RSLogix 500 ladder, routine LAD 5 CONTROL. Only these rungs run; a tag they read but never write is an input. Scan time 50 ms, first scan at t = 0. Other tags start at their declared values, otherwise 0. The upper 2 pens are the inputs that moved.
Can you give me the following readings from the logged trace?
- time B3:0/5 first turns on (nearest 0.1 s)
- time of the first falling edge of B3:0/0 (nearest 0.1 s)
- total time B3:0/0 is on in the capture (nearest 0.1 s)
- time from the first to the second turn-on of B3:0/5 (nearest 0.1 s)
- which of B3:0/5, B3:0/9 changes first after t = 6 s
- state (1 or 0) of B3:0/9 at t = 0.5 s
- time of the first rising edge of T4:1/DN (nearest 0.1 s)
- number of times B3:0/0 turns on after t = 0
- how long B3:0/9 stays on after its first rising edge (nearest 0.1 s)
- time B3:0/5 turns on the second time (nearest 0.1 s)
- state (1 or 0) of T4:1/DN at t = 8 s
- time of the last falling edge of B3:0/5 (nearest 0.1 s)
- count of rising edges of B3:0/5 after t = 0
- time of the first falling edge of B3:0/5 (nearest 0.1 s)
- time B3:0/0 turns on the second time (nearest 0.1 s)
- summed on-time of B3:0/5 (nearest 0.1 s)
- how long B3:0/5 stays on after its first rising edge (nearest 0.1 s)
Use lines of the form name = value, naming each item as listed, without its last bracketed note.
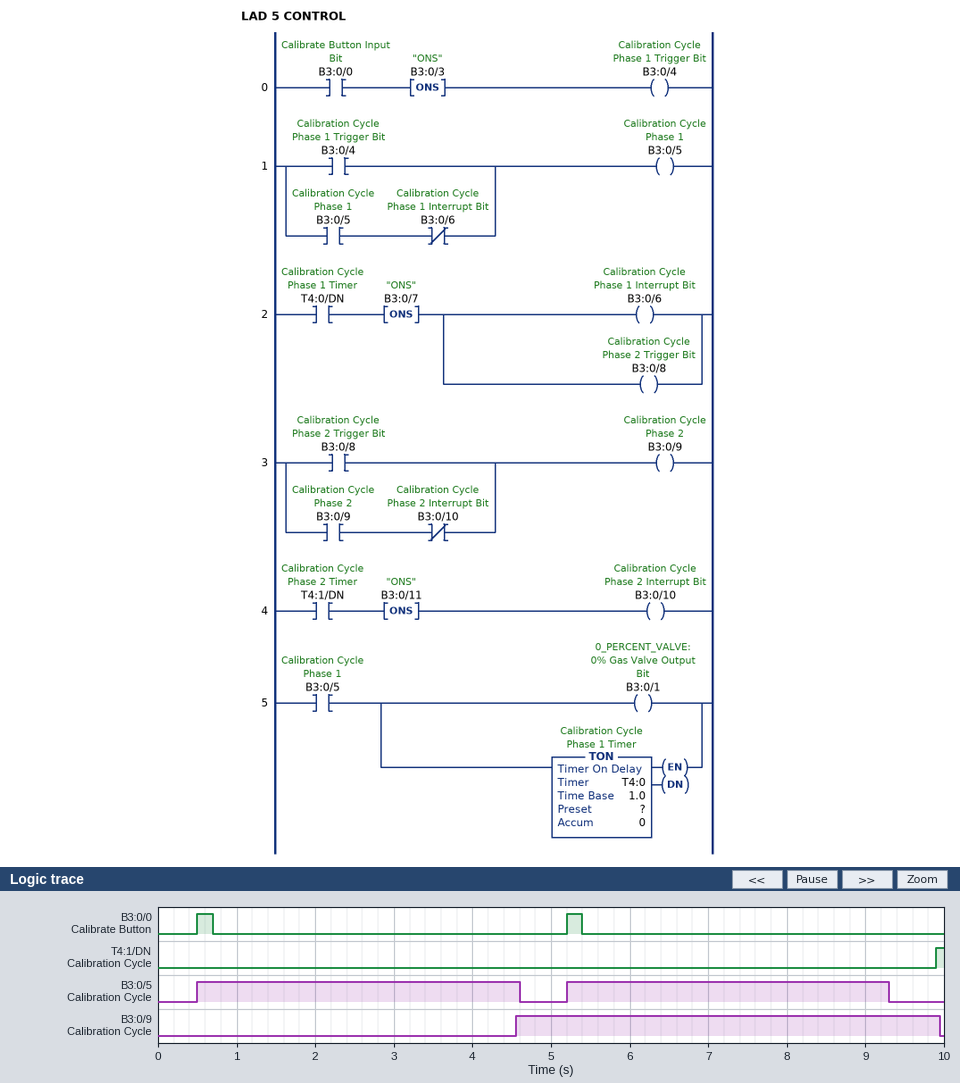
time B3:0/5 first turns on = 0.5 s
time of the first falling edge of B3:0/0 = 0.7 s
total time B3:0/0 is on in the capture = 0.4 s
time from the first to the second turn-on of B3:0/5 = 4.7 s
which of B3:0/5, B3:0/9 changes first after t = 6 s = B3:0/5
state (1 or 0) of B3:0/9 at t = 0.5 s = 0
time of the first rising edge of T4:1/DN = 9.9 s
number of times B3:0/0 turns on after t = 0 = 2
how long B3:0/9 stays on after its first rising edge = 5.4 s
time B3:0/5 turns on the second time = 5.2 s
state (1 or 0) of T4:1/DN at t = 8 s = 0
time of the last falling edge of B3:0/5 = 9.3 s
count of rising edges of B3:0/5 after t = 0 = 2
time of the first falling edge of B3:0/5 = 4.6 s
time B3:0/0 turns on the second time = 5.2 s
summed on-time of B3:0/5 = 8.2 s
how long B3:0/5 stays on after its first rising edge = 4.1 s
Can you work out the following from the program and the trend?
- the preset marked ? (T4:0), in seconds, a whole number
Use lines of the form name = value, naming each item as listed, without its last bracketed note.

the preset marked ? (T4:0), in seconds, a whole number = 4 s
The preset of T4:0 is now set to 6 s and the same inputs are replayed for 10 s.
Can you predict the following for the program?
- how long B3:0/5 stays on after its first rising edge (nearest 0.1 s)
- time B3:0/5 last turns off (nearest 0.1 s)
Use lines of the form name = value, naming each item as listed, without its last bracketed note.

how long B3:0/5 stays on after its first rising edge = 6.1 s
time B3:0/5 last turns off = 6.6 s
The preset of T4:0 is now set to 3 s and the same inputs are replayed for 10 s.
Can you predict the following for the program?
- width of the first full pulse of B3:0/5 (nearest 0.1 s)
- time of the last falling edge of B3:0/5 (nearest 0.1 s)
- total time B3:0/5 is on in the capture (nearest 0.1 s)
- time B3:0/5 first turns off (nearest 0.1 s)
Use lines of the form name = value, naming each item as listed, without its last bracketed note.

width of the first full pulse of B3:0/5 = 3.1 s
time of the last falling edge of B3:0/5 = 8.3 s
total time B3:0/5 is on in the capture = 6.2 s
time B3:0/5 first turns off = 3.6 s
